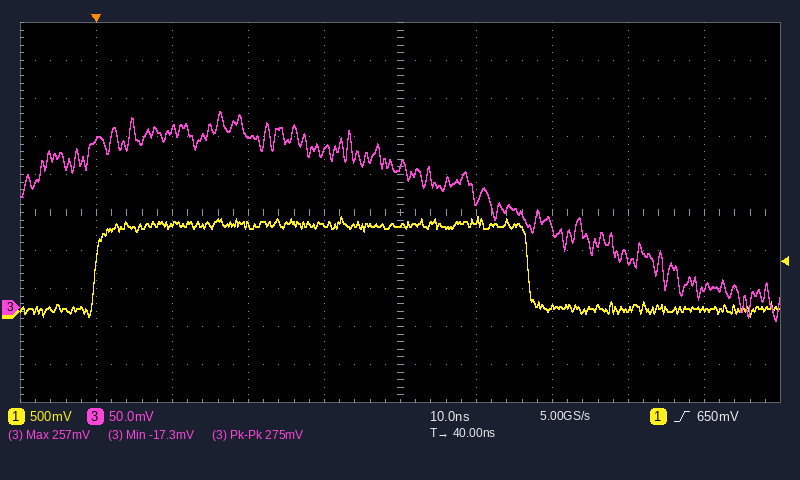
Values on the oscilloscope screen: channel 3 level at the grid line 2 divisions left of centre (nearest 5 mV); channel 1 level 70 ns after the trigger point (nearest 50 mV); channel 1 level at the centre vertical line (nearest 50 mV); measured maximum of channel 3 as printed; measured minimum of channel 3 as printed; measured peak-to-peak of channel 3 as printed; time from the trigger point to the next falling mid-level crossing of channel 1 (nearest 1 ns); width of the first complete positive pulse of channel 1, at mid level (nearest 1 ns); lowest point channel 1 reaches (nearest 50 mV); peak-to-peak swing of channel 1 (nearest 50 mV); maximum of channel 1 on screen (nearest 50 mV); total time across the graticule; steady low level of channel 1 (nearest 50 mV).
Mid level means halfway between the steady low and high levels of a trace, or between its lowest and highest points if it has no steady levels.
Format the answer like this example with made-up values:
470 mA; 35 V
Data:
225 mV; 50 mV; 1.15 V; 257 mV; -17.3 mV; 275 mV; 57 ns; 57 ns; -50 mV; 1.30 V; 1.25 V; 100 ns; 50 mV
